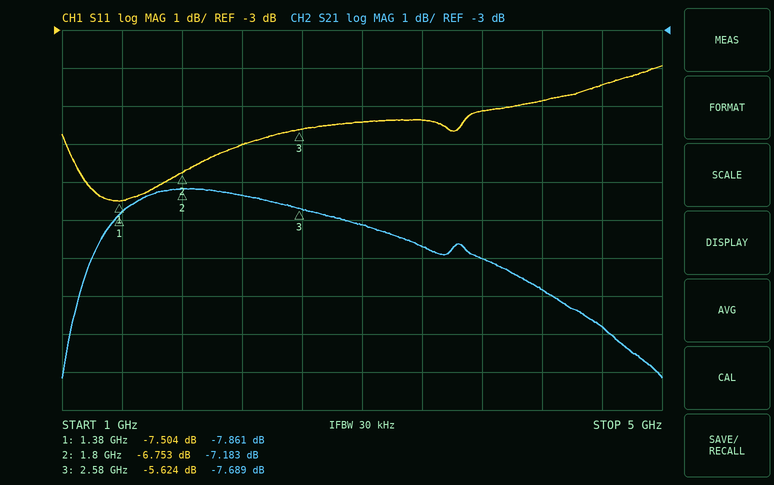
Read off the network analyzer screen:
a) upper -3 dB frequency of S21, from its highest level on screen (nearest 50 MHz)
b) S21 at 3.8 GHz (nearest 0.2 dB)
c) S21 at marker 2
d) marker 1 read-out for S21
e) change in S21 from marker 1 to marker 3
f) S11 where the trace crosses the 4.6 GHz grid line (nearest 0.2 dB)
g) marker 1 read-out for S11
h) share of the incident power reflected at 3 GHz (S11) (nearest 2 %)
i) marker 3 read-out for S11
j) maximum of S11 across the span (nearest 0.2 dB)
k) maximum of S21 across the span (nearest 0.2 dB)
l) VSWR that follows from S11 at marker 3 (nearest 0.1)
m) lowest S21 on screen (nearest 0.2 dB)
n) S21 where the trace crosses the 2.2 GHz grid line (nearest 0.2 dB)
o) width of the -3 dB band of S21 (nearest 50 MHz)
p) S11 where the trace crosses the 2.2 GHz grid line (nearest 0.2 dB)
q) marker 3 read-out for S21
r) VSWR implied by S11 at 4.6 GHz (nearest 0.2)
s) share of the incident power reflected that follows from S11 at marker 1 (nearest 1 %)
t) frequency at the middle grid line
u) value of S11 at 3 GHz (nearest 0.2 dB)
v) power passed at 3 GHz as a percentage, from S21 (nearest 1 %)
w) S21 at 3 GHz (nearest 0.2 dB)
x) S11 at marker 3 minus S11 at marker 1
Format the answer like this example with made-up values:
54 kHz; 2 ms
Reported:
4.35 GHz; -9.0 dB; -7.183 dB; -7.861 dB; 0.172 dB; -4.4 dB; -7.504 dB; 28 %; -5.624 dB; -4.0 dB; -7.2 dB; 3.2; -12.2 dB; -7.4 dB; 3.25 GHz; -6.0 dB; -7.689 dB; 4.0; 18 %; 3 GHz; -5.4 dB; 15 %; -8.2 dB; 1.880 dB
